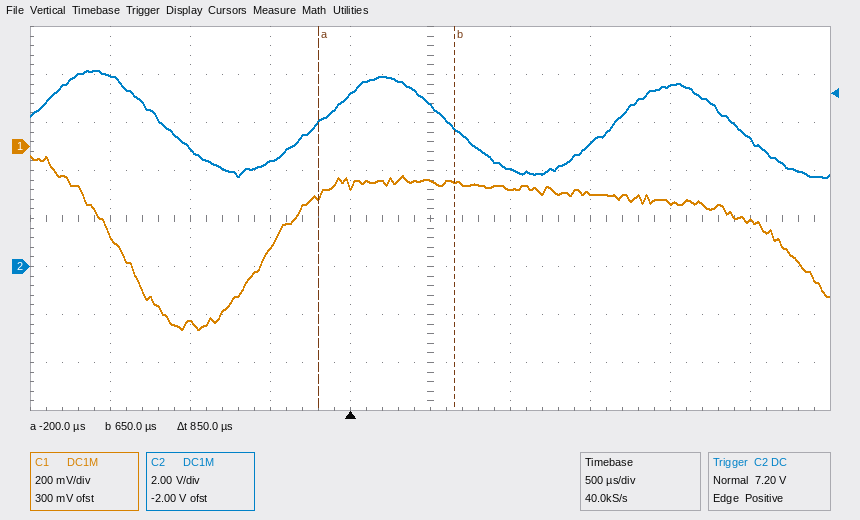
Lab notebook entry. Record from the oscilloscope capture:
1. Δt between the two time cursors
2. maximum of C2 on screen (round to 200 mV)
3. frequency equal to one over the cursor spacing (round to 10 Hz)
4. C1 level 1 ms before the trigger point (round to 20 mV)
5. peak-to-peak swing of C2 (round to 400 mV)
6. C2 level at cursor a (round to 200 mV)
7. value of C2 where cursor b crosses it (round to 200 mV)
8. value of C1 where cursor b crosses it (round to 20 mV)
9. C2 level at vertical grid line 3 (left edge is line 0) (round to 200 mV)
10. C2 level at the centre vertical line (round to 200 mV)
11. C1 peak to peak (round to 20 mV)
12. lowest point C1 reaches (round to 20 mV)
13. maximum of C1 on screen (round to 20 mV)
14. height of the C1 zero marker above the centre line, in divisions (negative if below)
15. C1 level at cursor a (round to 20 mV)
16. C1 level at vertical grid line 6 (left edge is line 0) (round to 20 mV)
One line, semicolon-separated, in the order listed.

850 µs; 8.2 V; 1.18 kHz; -740 mV; 4.4 V; 6.0 V; 5.8 V; -140 mV; 4.4 V; 6.8 V; 720 mV; -760 mV; -40 mV; +1.5 div; -200 mV; -180 mV
